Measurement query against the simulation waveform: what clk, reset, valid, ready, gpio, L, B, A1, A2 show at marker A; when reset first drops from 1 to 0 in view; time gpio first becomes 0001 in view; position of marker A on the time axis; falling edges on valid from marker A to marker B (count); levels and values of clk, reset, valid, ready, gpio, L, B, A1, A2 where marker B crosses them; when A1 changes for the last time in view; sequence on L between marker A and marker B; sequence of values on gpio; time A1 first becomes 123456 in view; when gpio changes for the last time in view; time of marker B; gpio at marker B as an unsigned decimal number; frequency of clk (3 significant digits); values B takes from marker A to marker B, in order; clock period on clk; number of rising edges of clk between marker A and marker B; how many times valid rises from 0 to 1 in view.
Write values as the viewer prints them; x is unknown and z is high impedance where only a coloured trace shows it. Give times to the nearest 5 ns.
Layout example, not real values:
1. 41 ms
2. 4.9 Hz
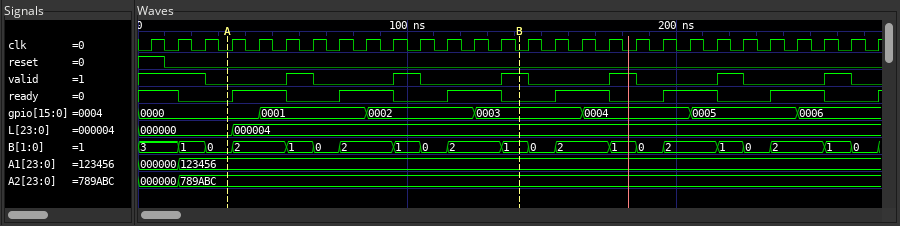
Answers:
1. clk=0, reset=0, valid=0, ready=0, gpio=0000, L=000000, B=0, A1=123456, A2=789ABC
2. 10 ns
3. 45 ns
4. 35 ns
5. 2
6. clk=0, reset=0, valid=1, ready=0, gpio=0003, L=000004, B=1, A1=123456, A2=789ABC
7. 15 ns
8. 000000, 000004
9. 0000, 0001, 0002, 0003, 0004, 0005, 0006
10. 15 ns
11. 245 ns
12. 140 ns
13. 3
14. 100 MHz
15. 0, 2, 1, 0, 2, 1, 0, 2, 1
16. 10 ns
17. 11
18. 6
